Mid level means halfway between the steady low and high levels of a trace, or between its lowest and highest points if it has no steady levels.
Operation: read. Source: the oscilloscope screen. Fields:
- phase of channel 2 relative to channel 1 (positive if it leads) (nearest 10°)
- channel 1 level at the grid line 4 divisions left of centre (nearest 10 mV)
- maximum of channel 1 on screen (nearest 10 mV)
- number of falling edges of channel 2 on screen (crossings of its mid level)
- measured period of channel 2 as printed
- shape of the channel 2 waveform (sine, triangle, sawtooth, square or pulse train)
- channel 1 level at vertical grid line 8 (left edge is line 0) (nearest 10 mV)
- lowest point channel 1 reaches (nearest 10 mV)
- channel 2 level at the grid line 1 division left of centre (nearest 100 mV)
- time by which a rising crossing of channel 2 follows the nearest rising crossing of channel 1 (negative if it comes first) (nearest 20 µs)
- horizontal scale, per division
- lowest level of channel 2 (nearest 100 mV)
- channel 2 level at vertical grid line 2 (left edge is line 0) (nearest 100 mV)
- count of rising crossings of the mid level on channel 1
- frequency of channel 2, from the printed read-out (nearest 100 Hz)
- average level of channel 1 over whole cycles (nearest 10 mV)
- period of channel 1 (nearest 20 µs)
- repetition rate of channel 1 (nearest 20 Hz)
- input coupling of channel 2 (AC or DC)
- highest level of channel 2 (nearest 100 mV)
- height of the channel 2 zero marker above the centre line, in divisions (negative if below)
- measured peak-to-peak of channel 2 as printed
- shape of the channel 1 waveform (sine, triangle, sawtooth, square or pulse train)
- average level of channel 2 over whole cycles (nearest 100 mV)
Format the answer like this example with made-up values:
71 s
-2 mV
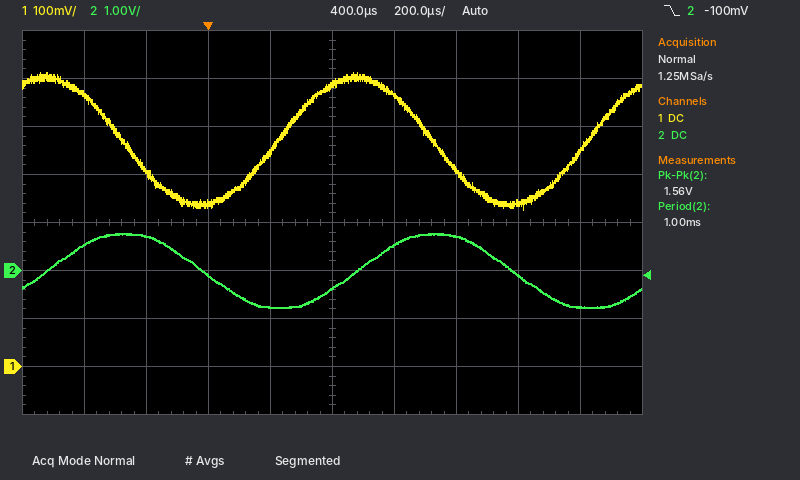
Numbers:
-90°
570 mV
610 mV
2
1.00 ms
sine
340 mV
330 mV
-800 mV
+260 µs
200 µs
-800 mV
700 mV
2
1.0 kHz
470 mV
1.00 ms
1.00 kHz
DC
800 mV
-1.0 div
1.56 V
sine
0.0 V
